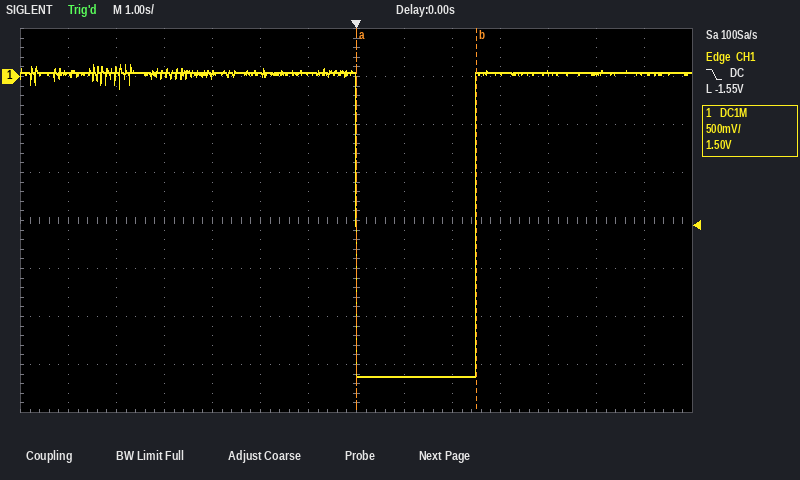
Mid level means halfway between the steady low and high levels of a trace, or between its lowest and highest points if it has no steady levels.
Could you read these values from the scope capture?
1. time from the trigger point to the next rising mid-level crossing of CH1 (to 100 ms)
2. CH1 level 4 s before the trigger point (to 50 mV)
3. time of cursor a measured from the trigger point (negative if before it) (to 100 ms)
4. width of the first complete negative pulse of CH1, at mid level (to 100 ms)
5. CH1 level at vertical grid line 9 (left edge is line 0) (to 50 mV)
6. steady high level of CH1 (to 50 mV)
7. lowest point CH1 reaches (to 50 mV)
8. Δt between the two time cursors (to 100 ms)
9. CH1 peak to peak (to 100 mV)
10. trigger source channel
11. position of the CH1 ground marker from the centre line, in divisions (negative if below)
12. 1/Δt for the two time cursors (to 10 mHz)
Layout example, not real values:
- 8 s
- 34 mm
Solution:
- 2.5 s
- 50 mV
- 0.0 s
- 2.5 s
- -3.10 V
- 50 mV
- -3.10 V
- 2.5 s
- 3.20 V
- CH1
- +3.0 div
- 400 mHz
